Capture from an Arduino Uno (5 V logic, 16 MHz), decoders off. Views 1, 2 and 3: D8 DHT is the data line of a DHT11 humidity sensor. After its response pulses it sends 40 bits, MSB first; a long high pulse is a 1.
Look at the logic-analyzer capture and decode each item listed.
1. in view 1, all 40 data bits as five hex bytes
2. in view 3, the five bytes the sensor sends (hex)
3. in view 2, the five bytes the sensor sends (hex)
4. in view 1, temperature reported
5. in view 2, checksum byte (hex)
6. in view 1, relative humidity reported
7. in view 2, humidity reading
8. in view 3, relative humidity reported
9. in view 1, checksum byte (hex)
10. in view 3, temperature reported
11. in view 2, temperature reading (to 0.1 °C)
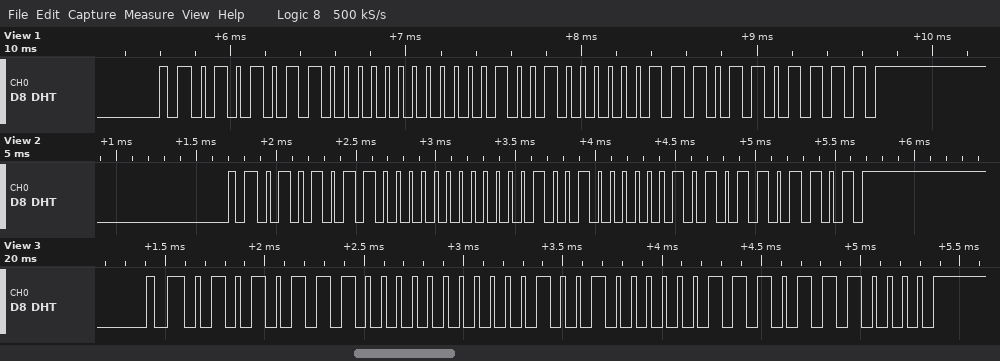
56 00 12 07 6F
57 00 12 07 70
56 00 12 05 6D
18.7 °C
0x6D
86 %
86 %
87 %
0x6F
18.7 °C
18.5 °C
